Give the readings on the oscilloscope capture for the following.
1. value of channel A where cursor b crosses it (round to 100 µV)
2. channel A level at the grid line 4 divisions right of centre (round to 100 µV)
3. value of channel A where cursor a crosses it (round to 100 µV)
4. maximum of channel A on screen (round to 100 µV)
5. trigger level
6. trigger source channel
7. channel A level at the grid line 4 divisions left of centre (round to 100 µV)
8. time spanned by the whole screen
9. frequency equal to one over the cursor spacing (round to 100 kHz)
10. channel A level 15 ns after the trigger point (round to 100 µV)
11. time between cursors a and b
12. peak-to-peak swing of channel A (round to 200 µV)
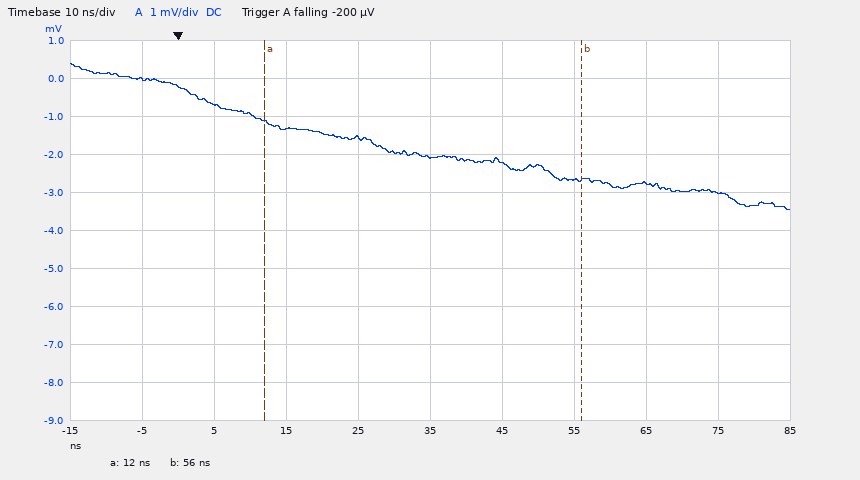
-2.7 mV
-3.0 mV
-1.1 mV
400 µV
-200 µV
channel A
0.0 mV
100 ns
22.7 MHz
-1.3 mV
44 ns
3.8 mV
